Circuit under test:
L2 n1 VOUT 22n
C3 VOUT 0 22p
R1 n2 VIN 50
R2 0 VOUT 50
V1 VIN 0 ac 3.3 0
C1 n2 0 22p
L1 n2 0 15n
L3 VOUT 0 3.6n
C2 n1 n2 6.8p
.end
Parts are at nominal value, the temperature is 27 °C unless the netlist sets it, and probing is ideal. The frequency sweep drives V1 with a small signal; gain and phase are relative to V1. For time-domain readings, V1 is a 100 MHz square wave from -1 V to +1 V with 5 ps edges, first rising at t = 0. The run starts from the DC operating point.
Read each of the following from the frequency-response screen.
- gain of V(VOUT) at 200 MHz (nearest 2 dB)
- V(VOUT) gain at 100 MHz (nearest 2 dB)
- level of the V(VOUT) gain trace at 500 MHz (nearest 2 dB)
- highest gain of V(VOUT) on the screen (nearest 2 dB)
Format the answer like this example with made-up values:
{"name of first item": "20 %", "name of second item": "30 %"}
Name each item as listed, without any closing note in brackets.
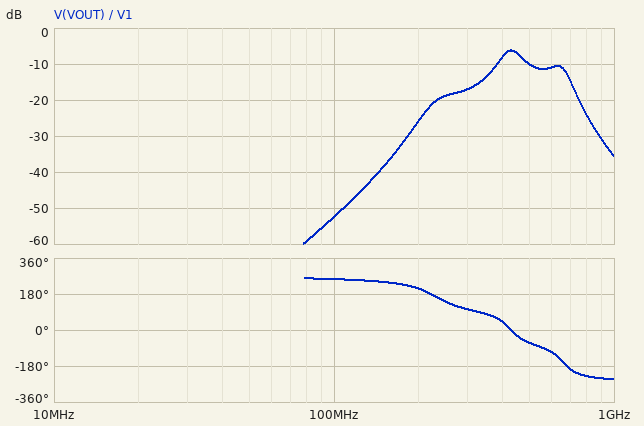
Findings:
{"gain of V(VOUT) at 200 MHz": "-26 dB", "V(VOUT) gain at 100 MHz": "-52 dB", "level of the V(VOUT) gain trace at 500 MHz": "-10 dB", "highest gain of V(VOUT) on the screen": "-6 dB"}
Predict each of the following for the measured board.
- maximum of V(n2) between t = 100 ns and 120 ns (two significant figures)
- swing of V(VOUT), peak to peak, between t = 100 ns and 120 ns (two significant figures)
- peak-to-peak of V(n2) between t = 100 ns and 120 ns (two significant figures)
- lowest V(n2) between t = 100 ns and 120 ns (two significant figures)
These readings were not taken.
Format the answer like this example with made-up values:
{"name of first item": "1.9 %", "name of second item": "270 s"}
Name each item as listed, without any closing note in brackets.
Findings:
{"maximum of V(n2) between t = 100 ns and 120 ns": "480 mV", "swing of V(VOUT), peak to peak, between t = 100 ns and 120 ns": "330 mV", "peak-to-peak of V(n2) between t = 100 ns and 120 ns": "970 mV", "lowest V(n2) between t = 100 ns and 120 ns": "-480 mV"}
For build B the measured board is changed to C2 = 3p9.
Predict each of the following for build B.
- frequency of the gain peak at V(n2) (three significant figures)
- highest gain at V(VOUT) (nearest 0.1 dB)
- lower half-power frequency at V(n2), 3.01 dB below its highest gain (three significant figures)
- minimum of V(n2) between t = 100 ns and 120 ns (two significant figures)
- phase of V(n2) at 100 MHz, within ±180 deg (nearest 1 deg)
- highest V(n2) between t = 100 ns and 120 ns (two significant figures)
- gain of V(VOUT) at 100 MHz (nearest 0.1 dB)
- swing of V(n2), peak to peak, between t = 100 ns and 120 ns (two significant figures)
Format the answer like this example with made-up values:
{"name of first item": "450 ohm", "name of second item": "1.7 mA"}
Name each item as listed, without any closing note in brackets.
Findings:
{"frequency of the gain peak at V(n2)": "249 MHz", "highest gain at V(VOUT)": "-7.5 dB", "lower half-power frequency at V(n2), 3.01 dB below its highest gain": "199 MHz", "minimum of V(n2) between t = 100 ns and 120 ns": "-570 mV", "phase of V(n2) at 100 MHz, within ±180 deg": "77 deg", "highest V(n2) between t = 100 ns and 120 ns": "570 mV", "gain of V(VOUT) at 100 MHz": "-57.8 dB", "swing of V(n2), peak to peak, between t = 100 ns and 120 ns": "1.1 V"}
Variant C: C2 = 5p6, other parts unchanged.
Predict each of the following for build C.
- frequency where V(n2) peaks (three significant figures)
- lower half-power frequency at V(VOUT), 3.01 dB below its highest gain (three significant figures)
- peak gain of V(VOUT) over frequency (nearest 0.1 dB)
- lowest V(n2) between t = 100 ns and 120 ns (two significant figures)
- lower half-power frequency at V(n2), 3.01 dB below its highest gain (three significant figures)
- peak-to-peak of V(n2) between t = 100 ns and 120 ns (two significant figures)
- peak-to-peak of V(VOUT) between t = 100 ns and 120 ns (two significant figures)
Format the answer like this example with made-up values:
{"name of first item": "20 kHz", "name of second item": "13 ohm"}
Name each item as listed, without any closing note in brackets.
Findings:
{"frequency where V(n2) peaks": "236 MHz", "lower half-power frequency at V(VOUT), 3.01 dB below its highest gain": "411 MHz", "peak gain of V(VOUT) over frequency": "-6.0 dB", "lowest V(n2) between t = 100 ns and 120 ns": "-530 mV", "lower half-power frequency at V(n2), 3.01 dB below its highest gain": "192 MHz", "peak-to-peak of V(n2) between t = 100 ns and 120 ns": "1.1 V", "peak-to-peak of V(VOUT) between t = 100 ns and 120 ns": "350 mV"}
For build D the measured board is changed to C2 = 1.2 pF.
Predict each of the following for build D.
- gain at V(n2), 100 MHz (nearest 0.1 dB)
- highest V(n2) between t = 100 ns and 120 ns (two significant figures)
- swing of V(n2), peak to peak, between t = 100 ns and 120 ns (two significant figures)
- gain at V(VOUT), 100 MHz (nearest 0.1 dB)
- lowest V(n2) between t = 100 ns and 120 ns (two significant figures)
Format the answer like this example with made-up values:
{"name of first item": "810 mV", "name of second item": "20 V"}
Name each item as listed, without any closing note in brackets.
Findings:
{"gain at V(n2), 100 MHz": "-13.4 dB", "highest V(n2) between t = 100 ns and 120 ns": "710 mV", "swing of V(n2), peak to peak, between t = 100 ns and 120 ns": "1.4 V", "gain at V(VOUT), 100 MHz": "-68.4 dB", "lowest V(n2) between t = 100 ns and 120 ns": "-710 mV"}
